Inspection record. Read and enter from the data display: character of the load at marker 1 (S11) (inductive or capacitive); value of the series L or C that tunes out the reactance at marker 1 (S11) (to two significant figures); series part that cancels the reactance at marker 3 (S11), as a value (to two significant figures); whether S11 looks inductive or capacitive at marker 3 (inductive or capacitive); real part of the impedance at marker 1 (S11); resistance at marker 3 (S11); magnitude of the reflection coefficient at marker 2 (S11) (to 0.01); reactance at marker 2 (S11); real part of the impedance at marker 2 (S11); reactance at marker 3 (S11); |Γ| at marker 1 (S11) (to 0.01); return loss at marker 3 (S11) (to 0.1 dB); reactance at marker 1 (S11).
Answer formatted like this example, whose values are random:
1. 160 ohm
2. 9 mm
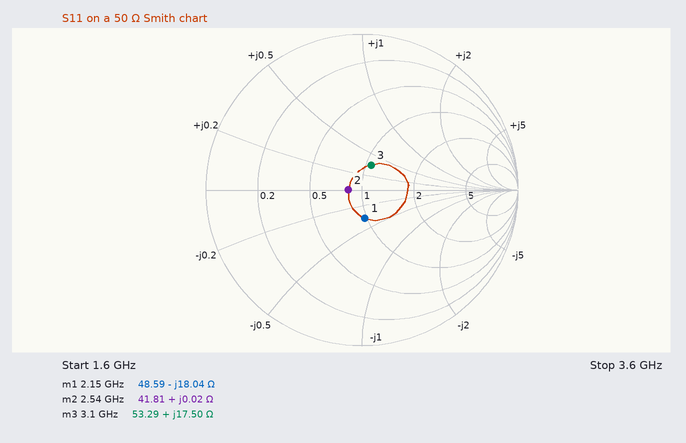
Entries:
1. capacitive
2. 1.3 nH
3. 2.9 pF
4. inductive
5. 48.59 Ω
6. 53.29 Ω
7. 0.09
8. +0.02 Ω
9. 41.81 Ω
10. +17.50 Ω
11. 0.18
12. 15.4 dB
13. -18.04 Ω
